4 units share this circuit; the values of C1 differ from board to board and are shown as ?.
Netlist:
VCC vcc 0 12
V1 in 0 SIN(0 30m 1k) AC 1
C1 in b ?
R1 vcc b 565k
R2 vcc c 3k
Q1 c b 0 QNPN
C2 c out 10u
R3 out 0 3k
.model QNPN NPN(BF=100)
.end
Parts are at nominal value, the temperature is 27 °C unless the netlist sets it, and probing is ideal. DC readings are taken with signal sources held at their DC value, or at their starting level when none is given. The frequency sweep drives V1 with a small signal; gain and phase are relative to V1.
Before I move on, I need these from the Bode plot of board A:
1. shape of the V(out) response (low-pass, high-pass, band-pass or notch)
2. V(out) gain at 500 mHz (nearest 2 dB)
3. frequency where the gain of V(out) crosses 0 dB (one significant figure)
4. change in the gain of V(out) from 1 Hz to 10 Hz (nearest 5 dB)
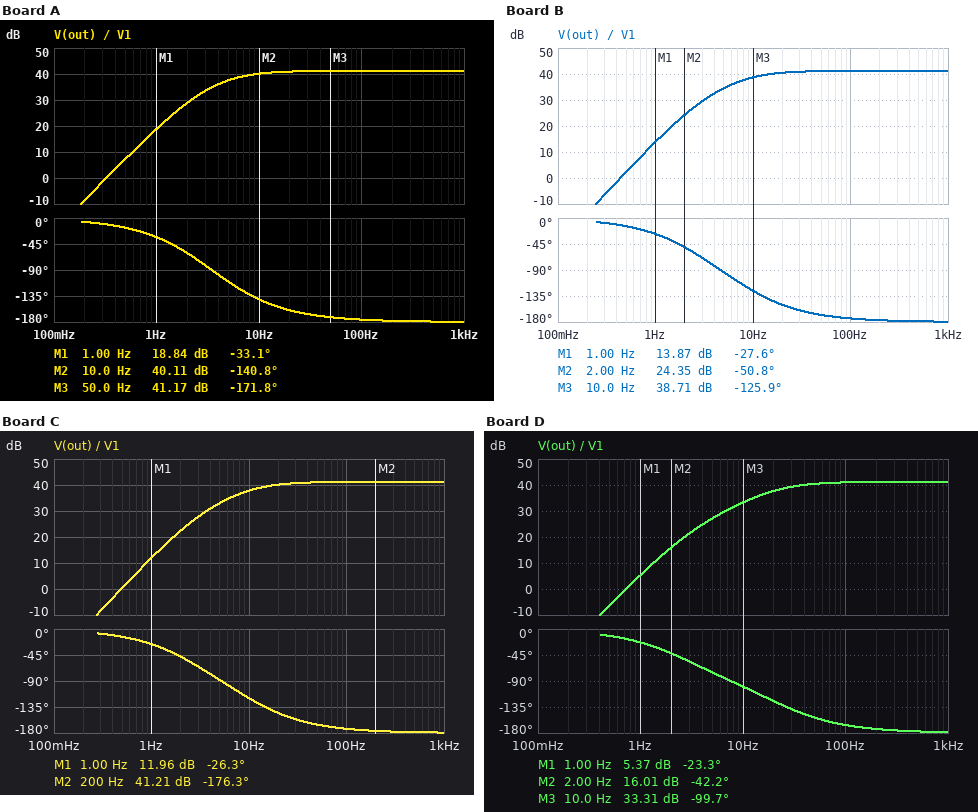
high-pass
8 dB
300 mHz
20 dB
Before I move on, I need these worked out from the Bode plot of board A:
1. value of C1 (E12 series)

27 µF
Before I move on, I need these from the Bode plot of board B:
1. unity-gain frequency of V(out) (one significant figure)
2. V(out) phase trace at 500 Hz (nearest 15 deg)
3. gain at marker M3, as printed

400 mHz
-180 deg
38.71 dB
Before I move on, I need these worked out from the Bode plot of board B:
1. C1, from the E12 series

15 µF
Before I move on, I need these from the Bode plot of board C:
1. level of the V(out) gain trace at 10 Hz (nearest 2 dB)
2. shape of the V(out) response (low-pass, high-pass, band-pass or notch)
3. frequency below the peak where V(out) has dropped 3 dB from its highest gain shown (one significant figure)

38 dB
high-pass
10 Hz
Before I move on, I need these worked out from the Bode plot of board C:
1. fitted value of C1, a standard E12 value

12 µF
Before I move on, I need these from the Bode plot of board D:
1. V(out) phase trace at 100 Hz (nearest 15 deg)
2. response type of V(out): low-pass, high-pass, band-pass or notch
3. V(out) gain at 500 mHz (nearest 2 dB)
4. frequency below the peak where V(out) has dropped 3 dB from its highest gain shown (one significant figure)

-165 deg
high-pass
-6 dB
20 Hz
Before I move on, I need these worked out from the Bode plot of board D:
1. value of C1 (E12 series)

5.6 µF
